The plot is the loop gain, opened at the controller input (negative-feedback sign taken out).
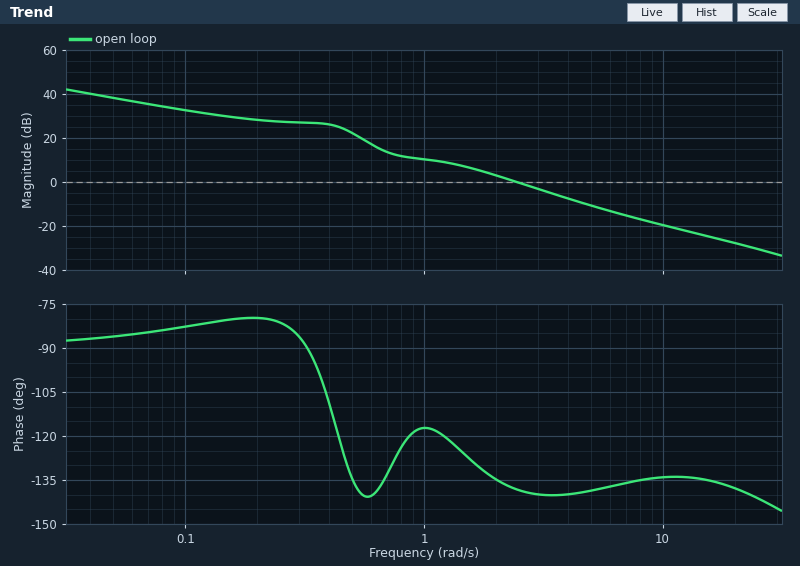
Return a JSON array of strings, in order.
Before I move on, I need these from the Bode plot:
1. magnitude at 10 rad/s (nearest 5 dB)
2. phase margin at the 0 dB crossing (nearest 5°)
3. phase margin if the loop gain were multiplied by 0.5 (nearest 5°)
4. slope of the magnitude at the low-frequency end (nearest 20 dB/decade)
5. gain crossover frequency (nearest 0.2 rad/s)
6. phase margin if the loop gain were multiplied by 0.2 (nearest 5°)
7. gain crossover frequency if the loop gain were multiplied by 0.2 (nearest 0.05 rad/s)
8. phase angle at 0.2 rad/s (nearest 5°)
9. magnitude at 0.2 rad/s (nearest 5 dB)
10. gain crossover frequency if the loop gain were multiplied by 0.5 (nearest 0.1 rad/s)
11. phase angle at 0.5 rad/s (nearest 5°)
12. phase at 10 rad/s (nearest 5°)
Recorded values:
["-20 dB", "40°", "50°", "-20 dB/decade", "2.4 rad/s", "45°", "0.70 rad/s", "-80°", "30 dB", "1.6 rad/s", "-135°", "-135°"]
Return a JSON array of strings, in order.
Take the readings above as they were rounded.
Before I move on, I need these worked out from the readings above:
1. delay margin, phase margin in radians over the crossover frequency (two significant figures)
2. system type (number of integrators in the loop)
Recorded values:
["0.29 s", "1"]
